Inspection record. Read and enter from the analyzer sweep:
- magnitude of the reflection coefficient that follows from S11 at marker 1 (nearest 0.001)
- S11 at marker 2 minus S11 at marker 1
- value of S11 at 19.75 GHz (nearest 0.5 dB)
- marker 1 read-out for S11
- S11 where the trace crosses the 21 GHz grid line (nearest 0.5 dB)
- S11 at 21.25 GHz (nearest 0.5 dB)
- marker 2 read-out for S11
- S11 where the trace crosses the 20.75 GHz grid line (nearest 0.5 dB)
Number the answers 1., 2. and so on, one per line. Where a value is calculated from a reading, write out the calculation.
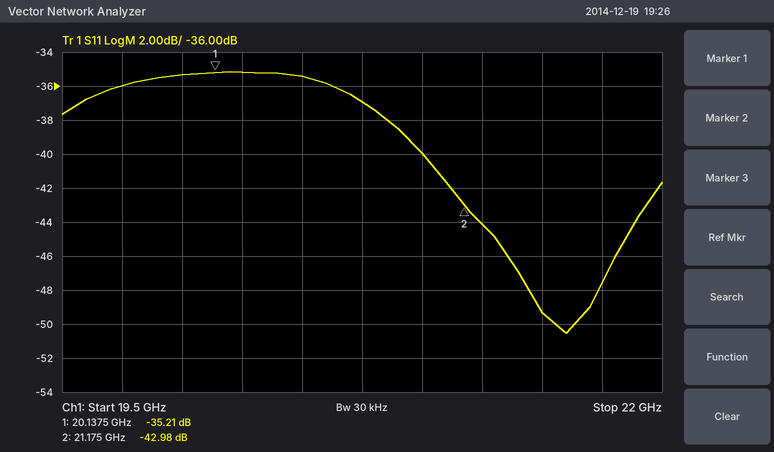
1. 10^(-35.21/20) ≈ 0.017
2. -42.98 − (-35.21) = -7.77 dB
3. -36.0 dB
4. -35.21 dB
5. -40.0 dB
6. -44.0 dB
7. -42.98 dB
8. -37.0 dB
